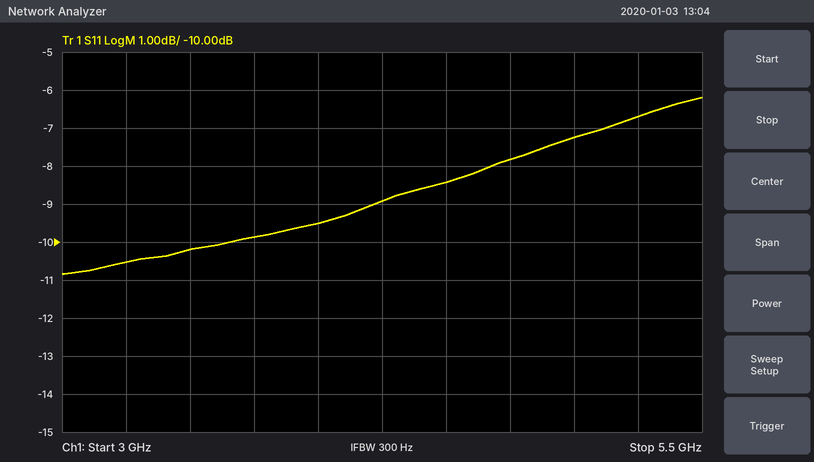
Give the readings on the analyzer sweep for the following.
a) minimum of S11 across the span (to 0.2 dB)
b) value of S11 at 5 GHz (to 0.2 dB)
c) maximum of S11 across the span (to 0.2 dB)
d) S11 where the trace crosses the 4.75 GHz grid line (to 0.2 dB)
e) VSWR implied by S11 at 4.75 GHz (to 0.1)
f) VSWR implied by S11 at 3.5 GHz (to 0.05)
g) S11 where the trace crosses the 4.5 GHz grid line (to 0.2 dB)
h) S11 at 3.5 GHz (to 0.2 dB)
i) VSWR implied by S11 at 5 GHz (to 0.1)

-10.8 dB
-7.2 dB
-6.2 dB
-7.8 dB
2.4
1.90
-8.4 dB
-10.2 dB
2.5
